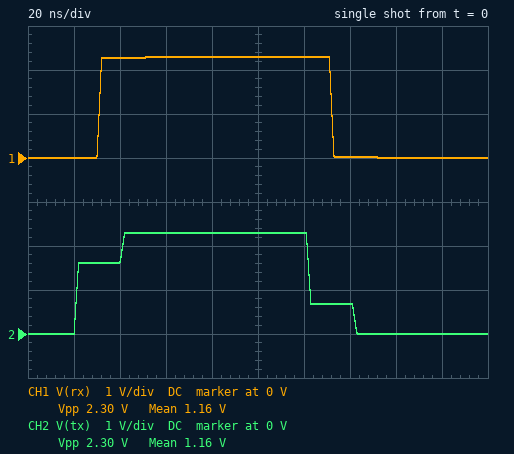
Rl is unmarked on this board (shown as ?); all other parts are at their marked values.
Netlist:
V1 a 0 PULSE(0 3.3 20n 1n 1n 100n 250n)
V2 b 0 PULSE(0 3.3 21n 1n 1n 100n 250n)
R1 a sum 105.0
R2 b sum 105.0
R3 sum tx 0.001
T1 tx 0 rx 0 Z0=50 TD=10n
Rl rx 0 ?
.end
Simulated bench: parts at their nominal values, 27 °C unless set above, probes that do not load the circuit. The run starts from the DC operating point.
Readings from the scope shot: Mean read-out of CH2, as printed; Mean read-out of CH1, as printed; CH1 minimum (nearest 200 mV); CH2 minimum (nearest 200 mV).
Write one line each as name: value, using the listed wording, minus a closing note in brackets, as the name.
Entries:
Mean read-out of CH2, as printed: 1.16 V
Mean read-out of CH1, as printed: 1.16 V
CH1 minimum: 0 V
CH2 minimum: 0 V
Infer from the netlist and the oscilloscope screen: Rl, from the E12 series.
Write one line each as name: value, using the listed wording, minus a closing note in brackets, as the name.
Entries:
Rl, from the E12 series: 120 Ω
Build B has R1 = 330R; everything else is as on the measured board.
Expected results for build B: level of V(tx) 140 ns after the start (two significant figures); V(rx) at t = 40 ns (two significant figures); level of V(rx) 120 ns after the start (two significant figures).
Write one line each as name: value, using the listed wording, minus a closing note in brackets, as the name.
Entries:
level of V(tx) 140 ns after the start: 710 mV
V(rx) at t = 40 ns: 1.8 V
level of V(rx) 120 ns after the start: 2.0 V
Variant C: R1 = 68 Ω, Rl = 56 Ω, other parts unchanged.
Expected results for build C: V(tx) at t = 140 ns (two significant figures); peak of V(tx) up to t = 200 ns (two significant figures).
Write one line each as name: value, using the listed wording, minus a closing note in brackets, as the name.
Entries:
V(tx) at t = 140 ns: 92 mV
peak of V(tx) up to t = 200 ns: 1.9 V
